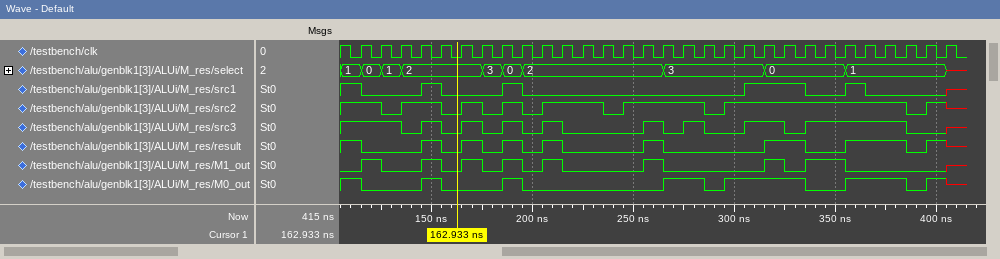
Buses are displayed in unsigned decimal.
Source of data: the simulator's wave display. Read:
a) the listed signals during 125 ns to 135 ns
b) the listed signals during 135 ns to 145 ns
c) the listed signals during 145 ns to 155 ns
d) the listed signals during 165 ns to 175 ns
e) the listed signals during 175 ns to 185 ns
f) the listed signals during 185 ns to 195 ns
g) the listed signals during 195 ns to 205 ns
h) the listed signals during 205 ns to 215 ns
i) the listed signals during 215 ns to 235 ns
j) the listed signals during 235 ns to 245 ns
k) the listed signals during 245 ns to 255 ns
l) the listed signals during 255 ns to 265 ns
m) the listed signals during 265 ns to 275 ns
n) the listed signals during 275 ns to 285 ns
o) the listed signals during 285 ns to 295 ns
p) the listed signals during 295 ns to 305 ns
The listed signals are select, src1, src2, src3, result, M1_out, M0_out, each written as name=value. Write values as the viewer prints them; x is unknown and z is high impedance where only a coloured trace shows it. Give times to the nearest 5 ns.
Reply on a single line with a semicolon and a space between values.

select=1, src1=0, src2=0, src3=1, result=0, M1_out=0, M0_out=0; select=2, src1=0, src2=1, src3=0, result=0, M1_out=0, M0_out=0; select=2, src1=1, src2=1, src3=1, result=1, M1_out=1, M0_out=1; select=2, src1=0, src2=1, src3=1, result=1, M1_out=1, M0_out=0; select=3, src1=0, src2=0, src3=0, result=0, M1_out=0, M0_out=0; select=0, src1=1, src2=1, src3=1, result=1, M1_out=1, M0_out=1; select=2, src1=0, src2=0, src3=0, result=0, M1_out=0, M0_out=0; select=2, src1=0, src2=1, src3=1, result=1, M1_out=1, M0_out=0; select=2, src1=0, src2=1, src3=0, result=0, M1_out=0, M0_out=0; select=2, src1=0, src2=0, src3=0, result=0, M1_out=0, M0_out=0; select=2, src1=0, src2=1, src3=0, result=0, M1_out=0, M0_out=0; select=2, src1=0, src2=1, src3=1, result=1, M1_out=1, M0_out=0; select=3, src1=0, src2=1, src3=0, result=0, M1_out=0, M0_out=1; select=3, src1=0, src2=1, src3=1, result=0, M1_out=0, M0_out=1; select=3, src1=0, src2=0, src3=0, result=0, M1_out=0, M0_out=0; select=3, src1=0, src2=1, src3=0, result=0, M1_out=0, M0_out=1
